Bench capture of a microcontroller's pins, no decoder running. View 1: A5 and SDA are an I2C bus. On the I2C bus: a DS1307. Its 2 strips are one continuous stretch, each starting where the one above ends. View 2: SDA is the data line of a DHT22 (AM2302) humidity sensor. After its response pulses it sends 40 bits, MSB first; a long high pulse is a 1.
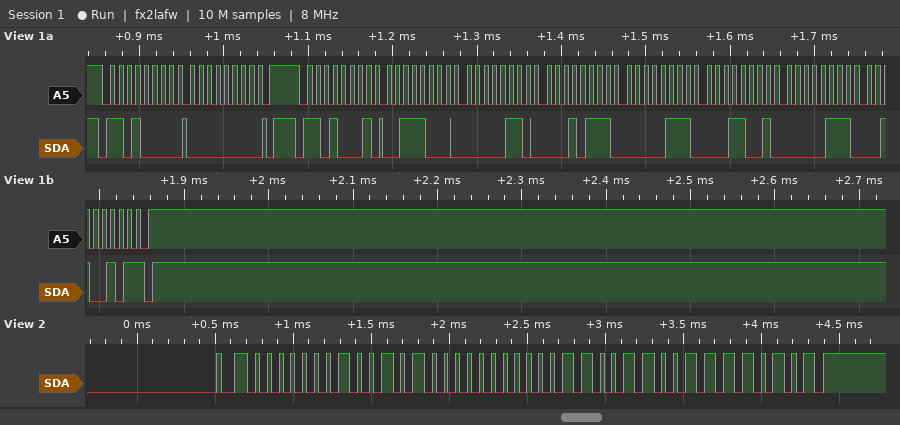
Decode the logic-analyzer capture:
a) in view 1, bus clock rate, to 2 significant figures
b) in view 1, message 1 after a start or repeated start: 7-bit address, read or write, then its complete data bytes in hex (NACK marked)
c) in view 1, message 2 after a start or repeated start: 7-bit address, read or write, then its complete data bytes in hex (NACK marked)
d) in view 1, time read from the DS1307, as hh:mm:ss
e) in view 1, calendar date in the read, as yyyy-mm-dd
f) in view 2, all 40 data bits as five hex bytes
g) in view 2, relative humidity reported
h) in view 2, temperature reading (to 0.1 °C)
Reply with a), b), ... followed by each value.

a) 100 kHz
b) 0x68 write: 00
c) 0x68 read: 38 06 17 07 19 07 25 NACK
d) 17:06:38
e) 2025-07-19
f) 01 28 00 CC F5
g) 29.6 %
h) 20.4 °C
